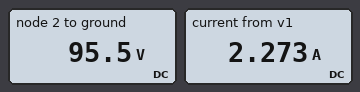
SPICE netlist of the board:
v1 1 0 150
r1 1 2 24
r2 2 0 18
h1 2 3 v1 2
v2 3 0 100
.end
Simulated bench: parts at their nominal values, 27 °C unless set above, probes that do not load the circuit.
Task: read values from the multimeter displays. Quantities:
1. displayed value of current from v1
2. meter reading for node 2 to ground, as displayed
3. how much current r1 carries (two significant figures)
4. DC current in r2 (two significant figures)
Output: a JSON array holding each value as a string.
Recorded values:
["2.273 A", "95.5 V", "2.3 A", "5.3 A"]
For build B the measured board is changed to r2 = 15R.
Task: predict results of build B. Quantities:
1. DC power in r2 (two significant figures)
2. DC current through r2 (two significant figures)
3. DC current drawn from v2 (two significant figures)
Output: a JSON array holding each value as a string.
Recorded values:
["610 W", "6.4 A", "4.1 A"]
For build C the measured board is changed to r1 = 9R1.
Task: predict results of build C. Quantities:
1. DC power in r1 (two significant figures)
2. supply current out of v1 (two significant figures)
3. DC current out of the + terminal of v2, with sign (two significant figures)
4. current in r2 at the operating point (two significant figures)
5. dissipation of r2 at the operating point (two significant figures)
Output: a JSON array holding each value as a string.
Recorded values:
["450 W", "7.0 A", "-2.3 A", "4.8 A", "410 W"]
